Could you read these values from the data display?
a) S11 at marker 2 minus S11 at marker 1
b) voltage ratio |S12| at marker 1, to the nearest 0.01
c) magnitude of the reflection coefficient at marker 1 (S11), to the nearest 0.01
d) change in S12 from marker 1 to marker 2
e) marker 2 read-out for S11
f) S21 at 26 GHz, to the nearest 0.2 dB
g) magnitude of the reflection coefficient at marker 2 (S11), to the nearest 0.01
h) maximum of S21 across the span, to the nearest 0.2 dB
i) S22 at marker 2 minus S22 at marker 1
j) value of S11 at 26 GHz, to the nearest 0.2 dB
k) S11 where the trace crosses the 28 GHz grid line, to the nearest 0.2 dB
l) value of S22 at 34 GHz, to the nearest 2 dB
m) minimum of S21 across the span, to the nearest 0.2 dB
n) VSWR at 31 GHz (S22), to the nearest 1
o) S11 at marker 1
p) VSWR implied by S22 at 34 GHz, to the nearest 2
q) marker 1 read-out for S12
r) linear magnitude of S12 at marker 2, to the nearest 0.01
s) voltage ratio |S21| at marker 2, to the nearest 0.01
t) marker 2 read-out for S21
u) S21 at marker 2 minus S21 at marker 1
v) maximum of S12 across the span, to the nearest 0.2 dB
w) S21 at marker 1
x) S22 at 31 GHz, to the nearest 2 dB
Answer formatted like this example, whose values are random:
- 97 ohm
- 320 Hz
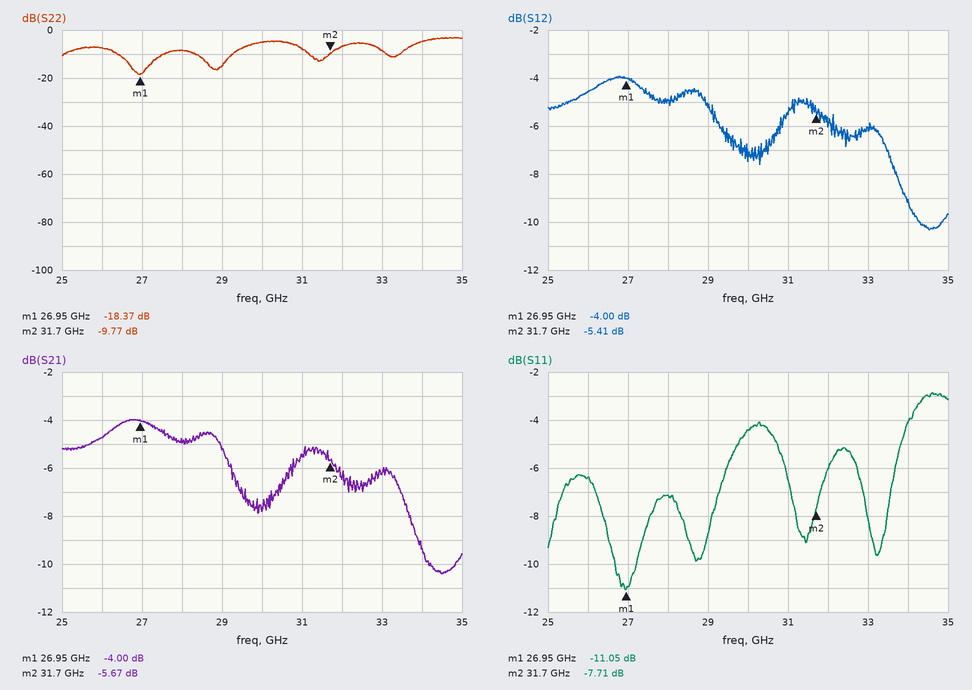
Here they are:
- 3.34 dB
- 0.63
- 0.28
- -1.41 dB
- -7.71 dB
- -4.8 dB
- 0.41
- -4.0 dB
- 8.60 dB
- -6.4 dB
- -7.2 dB
- -4 dB
- -10.4 dB
- 2
- -11.05 dB
- 4
- -4.00 dB
- 0.54
- 0.52
- -5.67 dB
- -1.67 dB
- -4.0 dB
- -4.00 dB
- -8 dB
